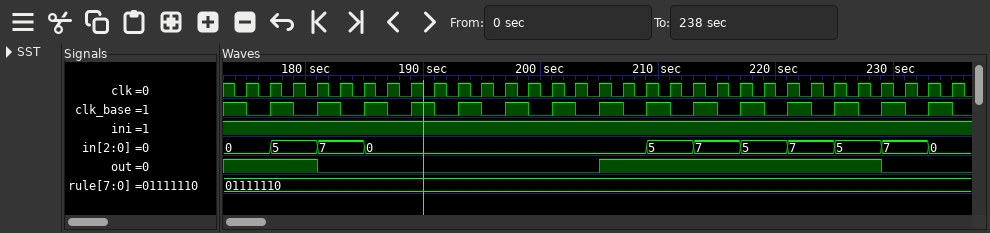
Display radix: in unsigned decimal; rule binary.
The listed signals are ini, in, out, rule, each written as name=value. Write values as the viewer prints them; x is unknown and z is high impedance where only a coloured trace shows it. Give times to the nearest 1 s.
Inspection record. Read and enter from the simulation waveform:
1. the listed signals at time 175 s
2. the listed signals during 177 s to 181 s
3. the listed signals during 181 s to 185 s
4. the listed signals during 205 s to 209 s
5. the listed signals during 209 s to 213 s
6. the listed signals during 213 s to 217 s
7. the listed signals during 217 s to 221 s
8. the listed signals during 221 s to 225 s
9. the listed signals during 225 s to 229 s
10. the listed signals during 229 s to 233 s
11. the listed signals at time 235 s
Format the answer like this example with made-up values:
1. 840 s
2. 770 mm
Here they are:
1. ini=1, in=0, out=1, rule=01111110
2. ini=1, in=5, out=1, rule=01111110
3. ini=1, in=7, out=0, rule=01111110
4. ini=1, in=0, out=1, rule=01111110
5. ini=1, in=5, out=1, rule=01111110
6. ini=1, in=7, out=1, rule=01111110
7. ini=1, in=5, out=1, rule=01111110
8. ini=1, in=7, out=1, rule=01111110
9. ini=1, in=5, out=1, rule=01111110
10. ini=1, in=7, out=0, rule=01111110
11. ini=1, in=0, out=0, rule=01111110
